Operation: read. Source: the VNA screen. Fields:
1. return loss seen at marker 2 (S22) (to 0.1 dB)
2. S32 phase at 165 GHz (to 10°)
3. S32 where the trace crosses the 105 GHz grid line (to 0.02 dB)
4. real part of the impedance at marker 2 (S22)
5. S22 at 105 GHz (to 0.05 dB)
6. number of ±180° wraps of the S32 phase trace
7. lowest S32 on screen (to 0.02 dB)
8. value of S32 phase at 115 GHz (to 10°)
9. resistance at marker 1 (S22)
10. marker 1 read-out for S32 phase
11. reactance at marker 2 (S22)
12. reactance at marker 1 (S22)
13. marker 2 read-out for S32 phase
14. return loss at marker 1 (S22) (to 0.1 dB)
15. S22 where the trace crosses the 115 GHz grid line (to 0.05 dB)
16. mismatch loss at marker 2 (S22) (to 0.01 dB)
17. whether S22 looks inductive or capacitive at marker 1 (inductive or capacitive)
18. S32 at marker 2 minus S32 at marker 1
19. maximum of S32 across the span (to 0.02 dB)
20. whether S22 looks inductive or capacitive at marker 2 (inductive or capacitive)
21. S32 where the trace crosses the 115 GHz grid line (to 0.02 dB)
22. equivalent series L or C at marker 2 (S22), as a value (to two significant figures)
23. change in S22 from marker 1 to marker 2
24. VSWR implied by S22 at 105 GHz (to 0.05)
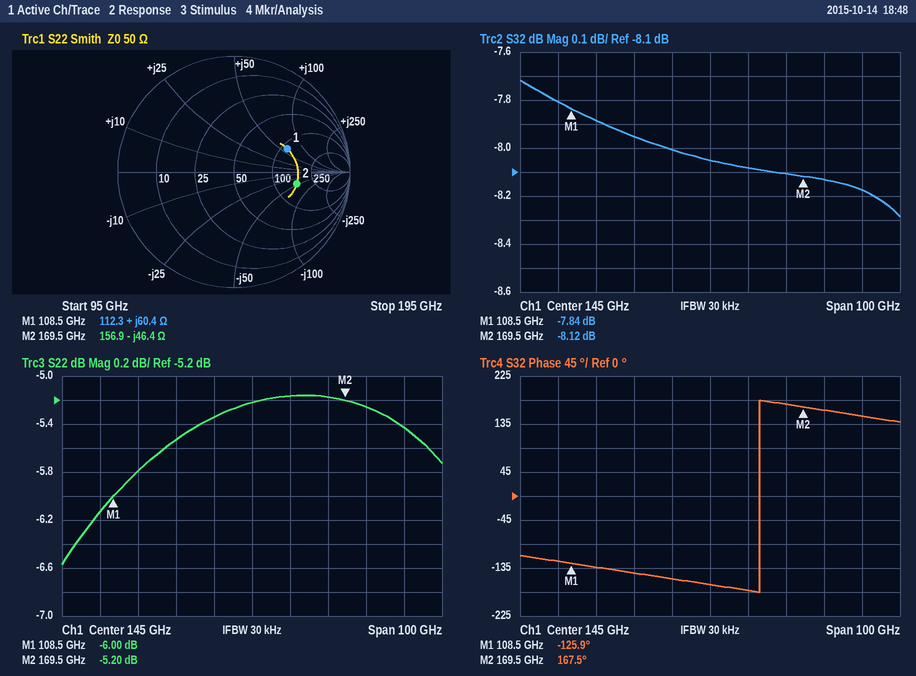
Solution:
5.2 dB
170°
-7.80 dB
156.9 Ω
-6.15 dB
1
-8.28 dB
-130°
112.3 Ω
-125.9°
-46.4 Ω
+60.4 Ω
167.5°
6.0 dB
-5.80 dB
1.56 dB
inductive
-0.28 dB
-7.72 dB
capacitive
-7.88 dB
20 fF
0.80 dB
2.95
